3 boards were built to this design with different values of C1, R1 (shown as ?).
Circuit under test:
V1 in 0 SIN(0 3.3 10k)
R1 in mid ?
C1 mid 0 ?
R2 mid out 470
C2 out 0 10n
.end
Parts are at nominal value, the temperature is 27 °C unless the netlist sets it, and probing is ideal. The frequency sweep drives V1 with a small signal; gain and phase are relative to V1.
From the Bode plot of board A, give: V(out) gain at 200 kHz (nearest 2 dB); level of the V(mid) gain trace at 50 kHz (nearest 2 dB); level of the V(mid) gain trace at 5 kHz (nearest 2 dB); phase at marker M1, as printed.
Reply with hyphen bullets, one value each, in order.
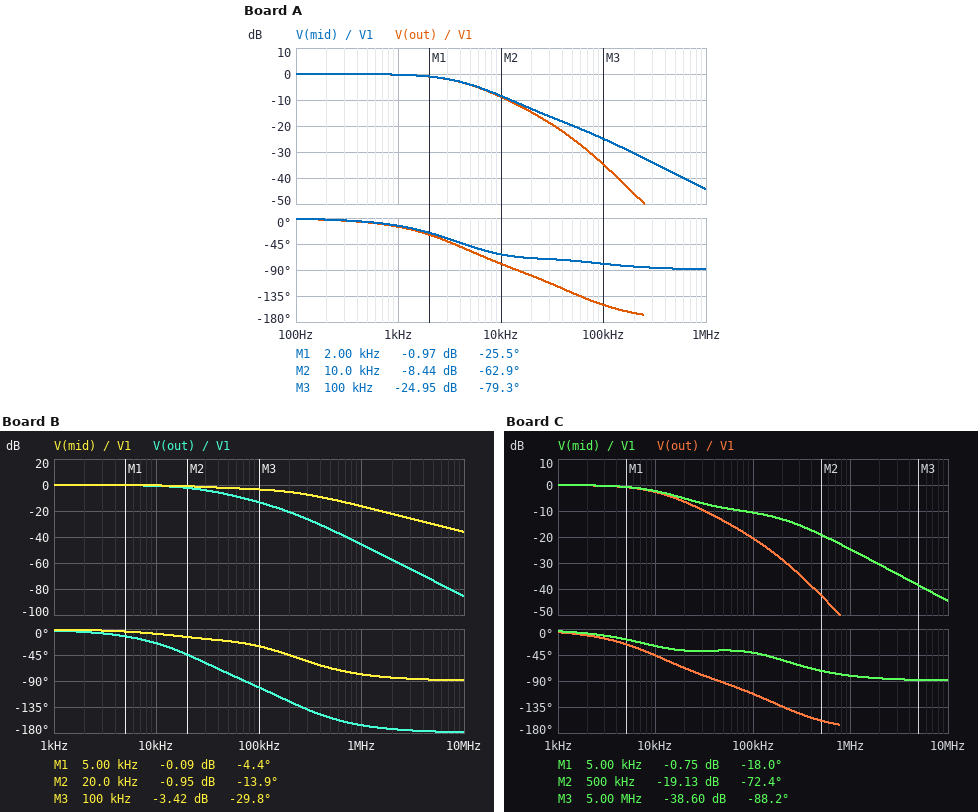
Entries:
- -46 dB
- -20 dB
- -4 dB
- -25.5 deg
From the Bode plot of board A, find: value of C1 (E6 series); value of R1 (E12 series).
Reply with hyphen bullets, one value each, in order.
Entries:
- 22 nF
- 1.2 kΩ
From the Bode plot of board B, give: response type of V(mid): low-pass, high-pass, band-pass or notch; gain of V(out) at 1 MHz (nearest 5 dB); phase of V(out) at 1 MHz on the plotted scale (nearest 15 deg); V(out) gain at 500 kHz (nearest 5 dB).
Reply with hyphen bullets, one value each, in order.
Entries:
- low-pass
- -45 dB
- -165 deg
- -35 dB
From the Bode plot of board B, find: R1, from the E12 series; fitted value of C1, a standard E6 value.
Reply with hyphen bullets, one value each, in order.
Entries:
- 150 Ω
- 6.8 nF
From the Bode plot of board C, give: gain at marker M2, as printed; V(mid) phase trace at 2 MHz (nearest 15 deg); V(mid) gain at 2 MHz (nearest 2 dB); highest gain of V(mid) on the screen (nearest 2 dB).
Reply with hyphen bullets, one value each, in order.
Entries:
- -19.13 dB
- -90 deg
- -30 dB
- 0 dB
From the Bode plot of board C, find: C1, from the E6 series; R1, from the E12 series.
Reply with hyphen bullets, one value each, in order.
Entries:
- 3.3 nF
- 820 Ω
